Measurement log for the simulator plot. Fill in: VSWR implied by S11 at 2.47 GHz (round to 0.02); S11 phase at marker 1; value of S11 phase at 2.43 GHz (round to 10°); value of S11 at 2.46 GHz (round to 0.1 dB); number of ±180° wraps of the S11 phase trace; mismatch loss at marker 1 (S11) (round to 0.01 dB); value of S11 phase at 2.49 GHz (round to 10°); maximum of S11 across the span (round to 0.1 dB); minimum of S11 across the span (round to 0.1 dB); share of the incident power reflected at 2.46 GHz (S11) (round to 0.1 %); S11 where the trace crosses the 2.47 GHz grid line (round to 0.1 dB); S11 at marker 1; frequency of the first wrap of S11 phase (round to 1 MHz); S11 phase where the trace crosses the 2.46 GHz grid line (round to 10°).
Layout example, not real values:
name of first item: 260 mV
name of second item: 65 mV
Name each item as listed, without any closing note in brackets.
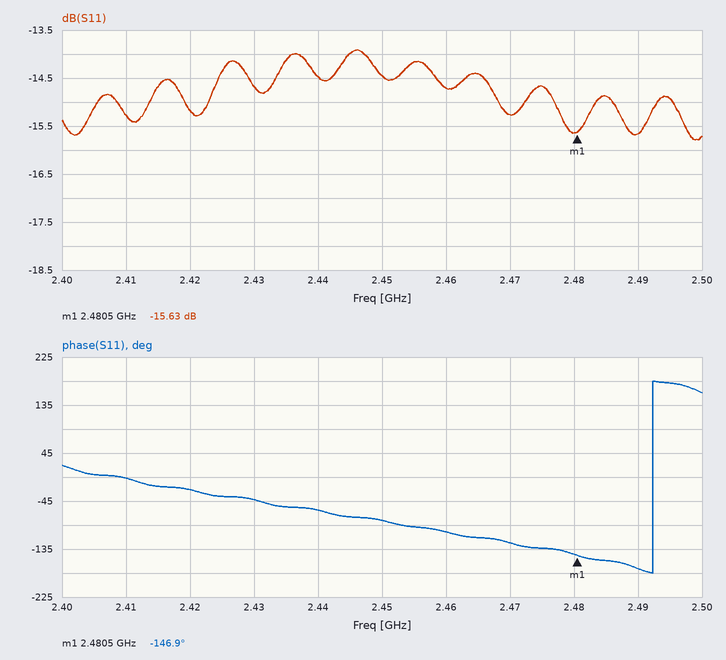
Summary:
VSWR implied by S11 at 2.47 GHz: 1.42
S11 phase at marker 1: -146.9°
value of S11 phase at 2.43 GHz: -40°
value of S11 at 2.46 GHz: -14.7 dB
number of ±180° wraps of the S11 phase trace: 1
mismatch loss at marker 1 (S11): 0.12 dB
value of S11 phase at 2.49 GHz: -170°
maximum of S11 across the span: -13.9 dB
minimum of S11 across the span: -15.8 dB
share of the incident power reflected at 2.46 GHz (S11): 3.4 %
S11 where the trace crosses the 2.47 GHz grid line: -15.3 dB
S11 at marker 1: -15.63 dB
frequency of the first wrap of S11 phase: 2.492 GHz
S11 phase where the trace crosses the 2.46 GHz grid line: -100°
